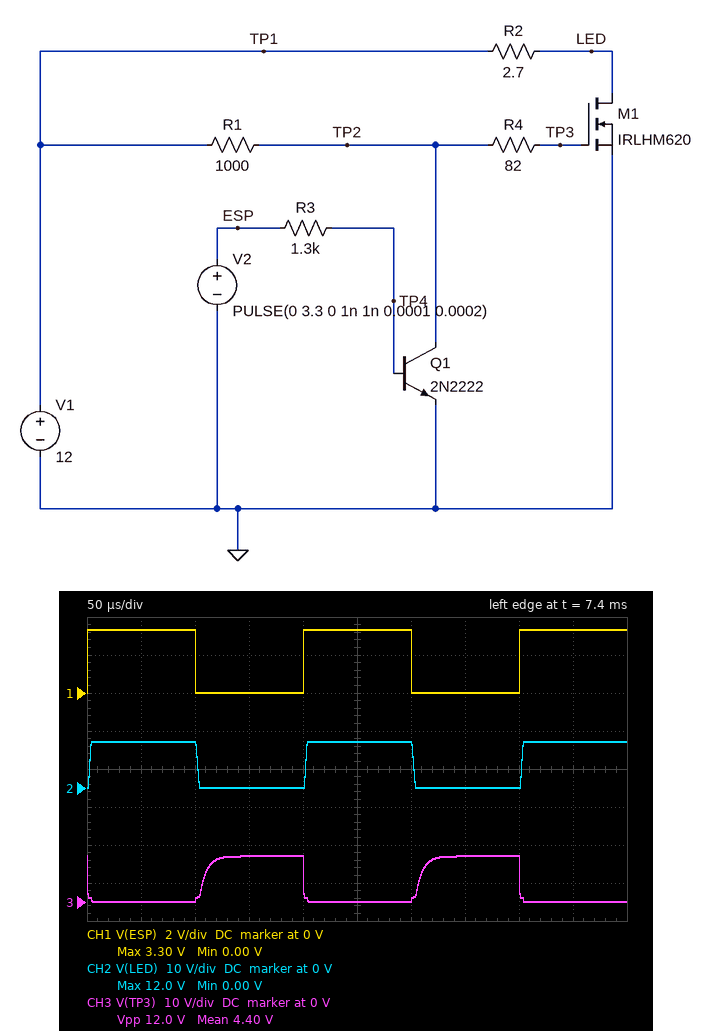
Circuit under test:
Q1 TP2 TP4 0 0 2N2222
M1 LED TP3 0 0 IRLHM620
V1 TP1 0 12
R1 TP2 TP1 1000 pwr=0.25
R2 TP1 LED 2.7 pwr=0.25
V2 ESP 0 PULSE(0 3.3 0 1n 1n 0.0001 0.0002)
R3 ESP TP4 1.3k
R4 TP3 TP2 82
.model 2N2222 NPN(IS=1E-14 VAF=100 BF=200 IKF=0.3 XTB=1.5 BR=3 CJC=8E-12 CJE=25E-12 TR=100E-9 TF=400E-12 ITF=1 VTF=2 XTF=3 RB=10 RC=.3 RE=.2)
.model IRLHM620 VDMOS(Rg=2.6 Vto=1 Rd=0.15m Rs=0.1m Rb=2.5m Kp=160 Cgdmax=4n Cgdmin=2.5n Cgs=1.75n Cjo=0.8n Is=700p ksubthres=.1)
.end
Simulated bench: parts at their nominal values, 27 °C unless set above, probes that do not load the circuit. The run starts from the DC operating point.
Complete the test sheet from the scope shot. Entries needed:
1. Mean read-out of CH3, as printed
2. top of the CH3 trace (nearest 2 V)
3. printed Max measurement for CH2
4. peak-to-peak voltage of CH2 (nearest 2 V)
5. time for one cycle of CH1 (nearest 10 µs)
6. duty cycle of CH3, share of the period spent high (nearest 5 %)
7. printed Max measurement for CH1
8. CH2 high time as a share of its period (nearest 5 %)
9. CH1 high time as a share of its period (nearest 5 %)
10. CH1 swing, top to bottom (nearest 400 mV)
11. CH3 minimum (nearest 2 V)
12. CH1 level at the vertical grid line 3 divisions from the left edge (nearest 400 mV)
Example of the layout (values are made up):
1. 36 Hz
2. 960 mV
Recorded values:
1. 4.40 V
2. 12 V
3. 12.0 V
4. 12 V
5. 200 µs
6. 45 %
7. 3.30 V
8. 50 %
9. 50 %
10. 3.2 V
11. 0 V
12. 0 V
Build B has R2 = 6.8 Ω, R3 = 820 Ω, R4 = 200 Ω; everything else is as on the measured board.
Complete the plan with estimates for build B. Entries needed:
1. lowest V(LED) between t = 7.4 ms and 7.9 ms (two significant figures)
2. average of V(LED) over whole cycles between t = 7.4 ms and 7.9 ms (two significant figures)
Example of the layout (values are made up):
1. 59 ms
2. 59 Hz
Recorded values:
1. 1.4 mV
2. 5.8 V
